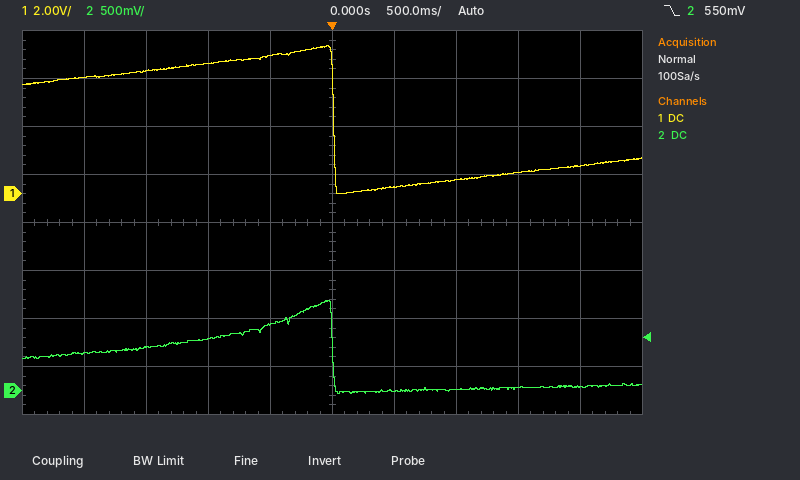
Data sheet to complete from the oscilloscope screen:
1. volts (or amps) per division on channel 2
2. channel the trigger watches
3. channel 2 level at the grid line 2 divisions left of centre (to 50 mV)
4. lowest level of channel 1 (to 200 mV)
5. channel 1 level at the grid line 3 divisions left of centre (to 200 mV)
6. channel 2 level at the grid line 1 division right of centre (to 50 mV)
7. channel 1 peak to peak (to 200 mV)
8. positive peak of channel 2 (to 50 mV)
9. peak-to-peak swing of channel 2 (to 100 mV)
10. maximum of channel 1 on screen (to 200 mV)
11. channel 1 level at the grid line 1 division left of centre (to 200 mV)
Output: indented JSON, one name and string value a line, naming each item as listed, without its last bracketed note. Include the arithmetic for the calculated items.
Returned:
{
  "volts (or amps) per division on channel 2": "500 mV",
  "channel the trigger watches": "channel 2",
  "channel 2 level at the grid line 2 divisions left of centre": "550 mV",
  "lowest level of channel 1": "0.0 V",
  "channel 1 level at the grid line 3 divisions left of centre": "5.2 V",
  "channel 2 level at the grid line 1 division right of centre": "0 mV",
  "channel 1 peak to peak": "6.2 V − (0.0 V) = 6.2 V",
  "positive peak of channel 2": "950 mV",
  "peak-to-peak swing of channel 2": "1.00 V",
  "maximum of channel 1 on screen": "6.2 V",
  "channel 1 level at the grid line 1 division left of centre": "5.8 V"
}
